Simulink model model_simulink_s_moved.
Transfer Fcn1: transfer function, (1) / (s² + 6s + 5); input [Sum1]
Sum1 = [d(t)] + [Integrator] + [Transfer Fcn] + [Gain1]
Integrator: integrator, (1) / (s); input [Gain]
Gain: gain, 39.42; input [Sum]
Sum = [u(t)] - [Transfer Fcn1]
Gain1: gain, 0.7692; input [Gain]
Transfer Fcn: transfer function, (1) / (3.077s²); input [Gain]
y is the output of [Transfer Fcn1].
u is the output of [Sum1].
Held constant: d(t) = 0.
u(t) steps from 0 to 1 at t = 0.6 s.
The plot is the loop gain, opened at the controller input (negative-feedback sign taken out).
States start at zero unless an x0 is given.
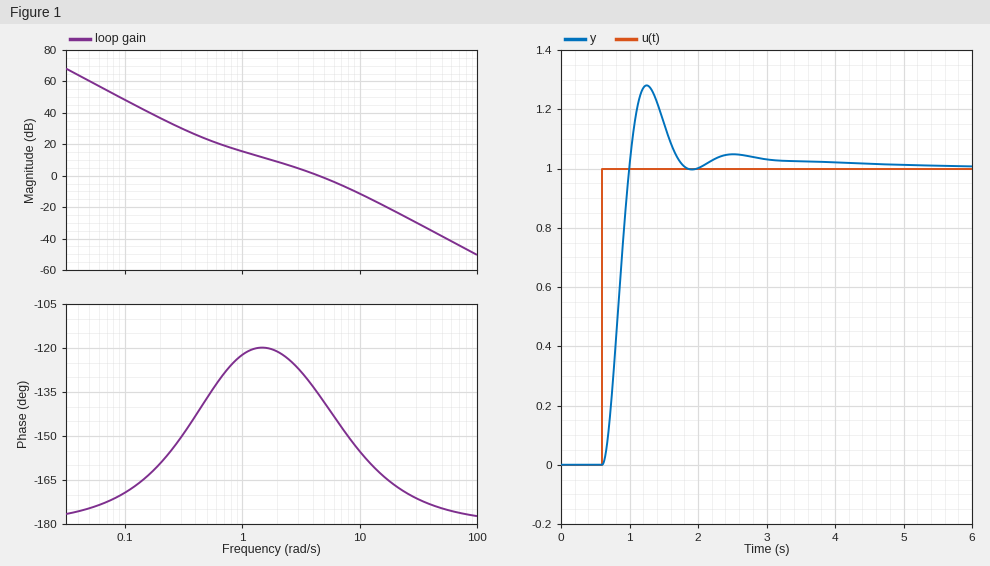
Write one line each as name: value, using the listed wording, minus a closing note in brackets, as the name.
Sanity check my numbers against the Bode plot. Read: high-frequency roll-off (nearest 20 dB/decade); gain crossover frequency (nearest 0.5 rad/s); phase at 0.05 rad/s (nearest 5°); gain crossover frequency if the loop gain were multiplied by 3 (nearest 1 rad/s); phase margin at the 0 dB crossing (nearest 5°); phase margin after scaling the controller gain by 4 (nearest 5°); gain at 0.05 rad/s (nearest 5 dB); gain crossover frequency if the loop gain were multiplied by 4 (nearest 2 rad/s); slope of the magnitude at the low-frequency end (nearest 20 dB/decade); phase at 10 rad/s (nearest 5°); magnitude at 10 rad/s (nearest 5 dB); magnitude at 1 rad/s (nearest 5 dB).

high-frequency roll-off: -40 dB/decade
gain crossover frequency: 4.5 rad/s
phase at 0.05 rad/s: -175°
gain crossover frequency if the loop gain were multiplied by 3: 9 rad/s
phase margin at the 0 dB crossing: 45°
phase margin after scaling the controller gain by 4: 25°
gain at 0.05 rad/s: 60 dB
gain crossover frequency if the loop gain were multiplied by 4: 10 rad/s
slope of the magnitude at the low-frequency end: -40 dB/decade
phase at 10 rad/s: -155°
magnitude at 10 rad/s: -10 dB
magnitude at 1 rad/s: 15 dB
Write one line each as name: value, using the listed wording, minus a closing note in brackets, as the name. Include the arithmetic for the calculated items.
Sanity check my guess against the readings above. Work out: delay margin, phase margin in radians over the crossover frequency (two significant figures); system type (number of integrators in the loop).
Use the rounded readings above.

delay margin, phase margin in radians over the crossover frequency: 45 × π / 180 / 4.5 = 0.17 s
system type: 2
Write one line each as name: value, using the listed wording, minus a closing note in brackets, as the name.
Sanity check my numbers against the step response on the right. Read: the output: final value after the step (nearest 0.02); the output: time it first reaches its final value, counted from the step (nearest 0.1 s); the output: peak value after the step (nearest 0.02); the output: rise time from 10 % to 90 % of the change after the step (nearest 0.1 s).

the output: final value after the step: 1.00
the output: time it first reaches its final value, counted from the step: 0.4 s
the output: peak value after the step: 1.28
the output: rise time from 10 % to 90 % of the change after the step: 0.3 s
